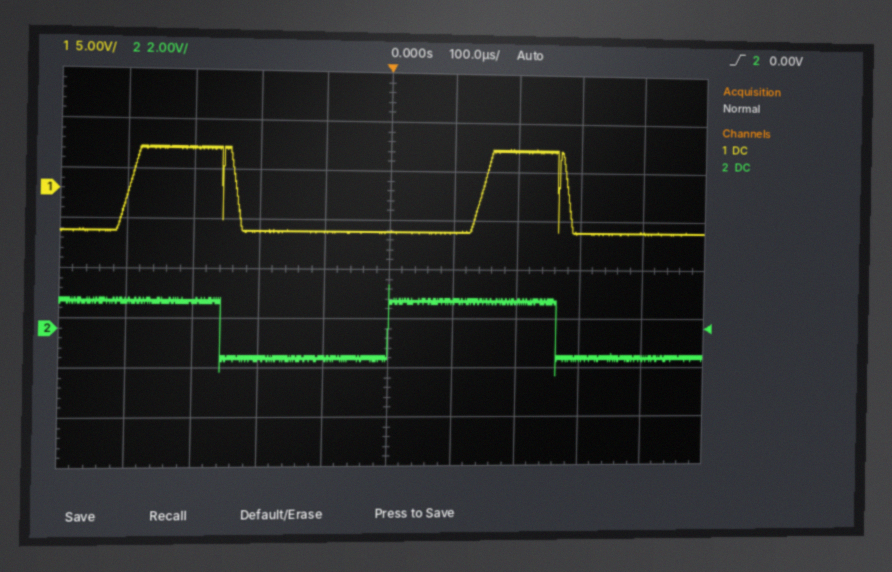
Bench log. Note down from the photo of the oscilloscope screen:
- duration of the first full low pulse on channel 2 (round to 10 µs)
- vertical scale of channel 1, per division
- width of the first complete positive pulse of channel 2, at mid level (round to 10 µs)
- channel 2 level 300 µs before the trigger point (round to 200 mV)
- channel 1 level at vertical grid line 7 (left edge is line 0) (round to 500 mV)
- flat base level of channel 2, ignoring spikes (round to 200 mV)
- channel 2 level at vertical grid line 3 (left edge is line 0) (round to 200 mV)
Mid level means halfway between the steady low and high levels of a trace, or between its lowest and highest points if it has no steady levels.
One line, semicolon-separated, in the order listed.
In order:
260 µs; 5 V; 260 µs; 1.0 V; 4.0 V; -1.2 V; -1.2 V
